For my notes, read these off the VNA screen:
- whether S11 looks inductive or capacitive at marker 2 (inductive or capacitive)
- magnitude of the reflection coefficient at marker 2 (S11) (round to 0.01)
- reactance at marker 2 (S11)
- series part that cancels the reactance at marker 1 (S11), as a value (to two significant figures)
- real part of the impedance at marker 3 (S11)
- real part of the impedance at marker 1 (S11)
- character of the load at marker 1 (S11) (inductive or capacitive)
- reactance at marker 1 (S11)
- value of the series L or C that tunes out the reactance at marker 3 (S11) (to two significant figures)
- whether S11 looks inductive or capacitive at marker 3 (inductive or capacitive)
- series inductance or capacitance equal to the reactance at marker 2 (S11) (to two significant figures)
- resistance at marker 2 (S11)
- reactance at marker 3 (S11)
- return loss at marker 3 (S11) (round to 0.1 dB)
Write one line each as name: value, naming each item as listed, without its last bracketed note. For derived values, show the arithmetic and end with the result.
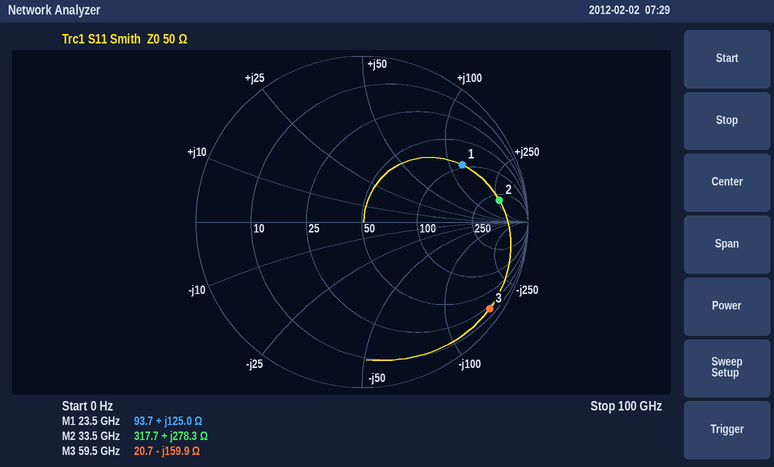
whether S11 looks inductive or capacitive at marker 2: inductive
magnitude of the reflection coefficient at marker 2 (S11): 0.84
reactance at marker 2: +278.3 Ω
series part that cancels the reactance at marker 1 (S11), as a value: C = 1/(2π × 23.5 GHz × 125 Ω) ≈ 54 fF
real part of the impedance at marker 3: 20.7 Ω
real part of the impedance at marker 1: 93.7 Ω
character of the load at marker 1 (S11): inductive
reactance at marker 1: +125.0 Ω
value of the series L or C that tunes out the reactance at marker 3 (S11): L = 159.9 Ω/(2π × 59.5 GHz) ≈ 428 pH, so 430 pH to two significant figures
whether S11 looks inductive or capacitive at marker 3: capacitive
series inductance or capacitance equal to the reactance at marker 2 (S11): L = 278.3 Ω/(2π × 33.5 GHz) ≈ 1.3 nH
resistance at marker 2: 317.7 Ω
reactance at marker 3: -159.9 Ω
return loss at marker 3 (S11): 0.6 dB
